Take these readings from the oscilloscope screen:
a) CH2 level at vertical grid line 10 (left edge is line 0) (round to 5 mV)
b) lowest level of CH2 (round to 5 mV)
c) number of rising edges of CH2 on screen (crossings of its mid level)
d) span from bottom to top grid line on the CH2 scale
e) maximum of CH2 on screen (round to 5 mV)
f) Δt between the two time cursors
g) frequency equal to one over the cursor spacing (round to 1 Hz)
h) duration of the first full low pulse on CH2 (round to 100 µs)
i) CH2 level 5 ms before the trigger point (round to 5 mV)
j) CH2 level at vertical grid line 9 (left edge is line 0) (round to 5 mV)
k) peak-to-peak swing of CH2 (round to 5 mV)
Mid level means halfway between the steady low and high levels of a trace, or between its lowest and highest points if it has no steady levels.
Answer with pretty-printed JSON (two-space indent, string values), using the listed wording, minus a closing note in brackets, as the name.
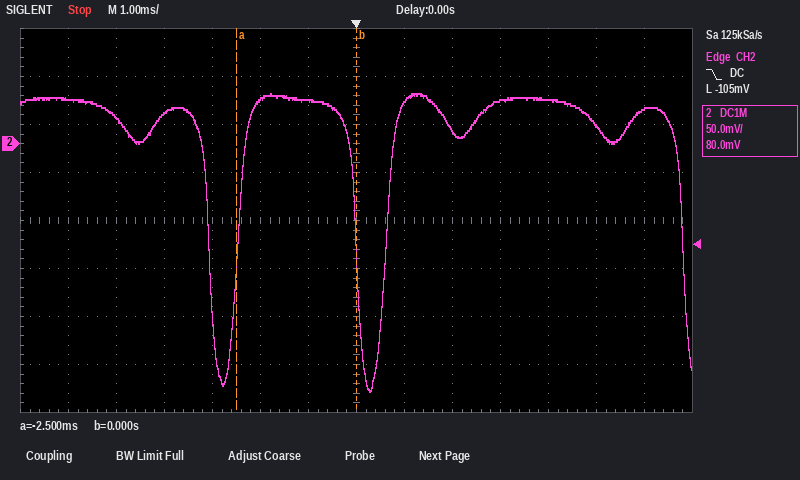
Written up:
{
  "CH2 level at vertical grid line 10 (left edge is line 0)": "45 mV",
  "lowest level of CH2": "-260 mV",
  "number of rising edges of CH2 on screen": "2",
  "span from bottom to top grid line on the CH2 scale": "400 mV",
  "maximum of CH2 on screen": "50 mV",
  "Δt between the two time cursors": "2.5 ms",
  "frequency equal to one over the cursor spacing": "400 Hz",
  "duration of the first full low pulse on CH2": "600 µs",
  "CH2 level 5 ms before the trigger point": "30 mV",
  "CH2 level at vertical grid line 9 (left edge is line 0)": "15 mV",
  "peak-to-peak swing of CH2": "310 mV"
}
